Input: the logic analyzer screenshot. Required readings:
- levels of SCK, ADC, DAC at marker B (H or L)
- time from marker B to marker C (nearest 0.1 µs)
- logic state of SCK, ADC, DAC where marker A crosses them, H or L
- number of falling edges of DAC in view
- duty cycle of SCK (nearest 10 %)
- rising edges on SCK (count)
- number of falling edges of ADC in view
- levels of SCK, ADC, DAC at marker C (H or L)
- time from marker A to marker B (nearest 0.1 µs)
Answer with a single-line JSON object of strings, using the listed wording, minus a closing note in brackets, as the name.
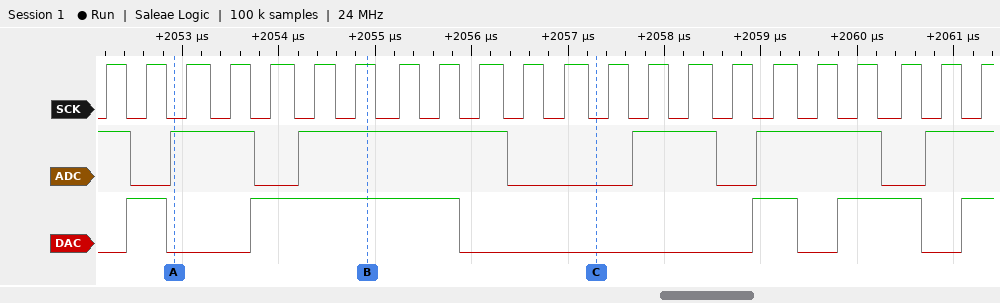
{"levels of SCK, ADC, DAC at marker B": "SCK=H, ADC=H, DAC=H", "time from marker B to marker C": "2.4 µs", "logic state of SCK, ADC, DAC where marker A crosses them, H or L": "SCK=L, ADC=H, DAC=L", "number of falling edges of DAC in view": "4", "duty cycle of SCK": "50 %", "rising edges on SCK": "22", "number of falling edges of ADC in view": "5", "levels of SCK, ADC, DAC at marker C": "SCK=L, ADC=L, DAC=L", "time from marker A to marker B": "2 µs"}
